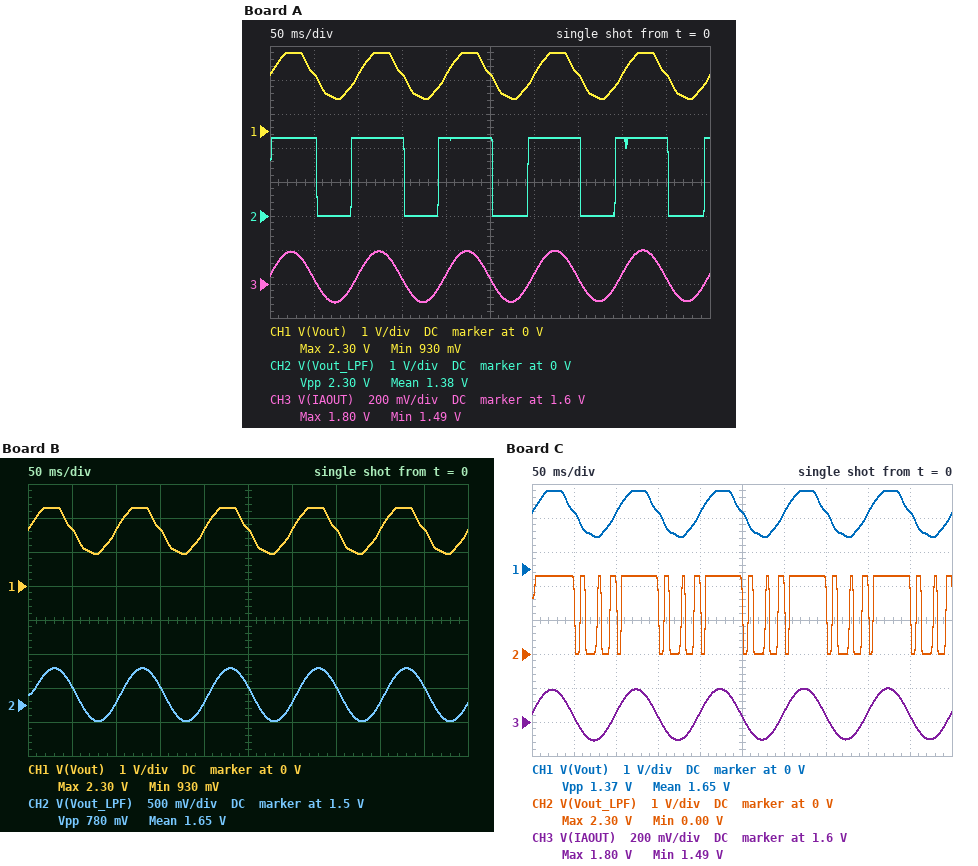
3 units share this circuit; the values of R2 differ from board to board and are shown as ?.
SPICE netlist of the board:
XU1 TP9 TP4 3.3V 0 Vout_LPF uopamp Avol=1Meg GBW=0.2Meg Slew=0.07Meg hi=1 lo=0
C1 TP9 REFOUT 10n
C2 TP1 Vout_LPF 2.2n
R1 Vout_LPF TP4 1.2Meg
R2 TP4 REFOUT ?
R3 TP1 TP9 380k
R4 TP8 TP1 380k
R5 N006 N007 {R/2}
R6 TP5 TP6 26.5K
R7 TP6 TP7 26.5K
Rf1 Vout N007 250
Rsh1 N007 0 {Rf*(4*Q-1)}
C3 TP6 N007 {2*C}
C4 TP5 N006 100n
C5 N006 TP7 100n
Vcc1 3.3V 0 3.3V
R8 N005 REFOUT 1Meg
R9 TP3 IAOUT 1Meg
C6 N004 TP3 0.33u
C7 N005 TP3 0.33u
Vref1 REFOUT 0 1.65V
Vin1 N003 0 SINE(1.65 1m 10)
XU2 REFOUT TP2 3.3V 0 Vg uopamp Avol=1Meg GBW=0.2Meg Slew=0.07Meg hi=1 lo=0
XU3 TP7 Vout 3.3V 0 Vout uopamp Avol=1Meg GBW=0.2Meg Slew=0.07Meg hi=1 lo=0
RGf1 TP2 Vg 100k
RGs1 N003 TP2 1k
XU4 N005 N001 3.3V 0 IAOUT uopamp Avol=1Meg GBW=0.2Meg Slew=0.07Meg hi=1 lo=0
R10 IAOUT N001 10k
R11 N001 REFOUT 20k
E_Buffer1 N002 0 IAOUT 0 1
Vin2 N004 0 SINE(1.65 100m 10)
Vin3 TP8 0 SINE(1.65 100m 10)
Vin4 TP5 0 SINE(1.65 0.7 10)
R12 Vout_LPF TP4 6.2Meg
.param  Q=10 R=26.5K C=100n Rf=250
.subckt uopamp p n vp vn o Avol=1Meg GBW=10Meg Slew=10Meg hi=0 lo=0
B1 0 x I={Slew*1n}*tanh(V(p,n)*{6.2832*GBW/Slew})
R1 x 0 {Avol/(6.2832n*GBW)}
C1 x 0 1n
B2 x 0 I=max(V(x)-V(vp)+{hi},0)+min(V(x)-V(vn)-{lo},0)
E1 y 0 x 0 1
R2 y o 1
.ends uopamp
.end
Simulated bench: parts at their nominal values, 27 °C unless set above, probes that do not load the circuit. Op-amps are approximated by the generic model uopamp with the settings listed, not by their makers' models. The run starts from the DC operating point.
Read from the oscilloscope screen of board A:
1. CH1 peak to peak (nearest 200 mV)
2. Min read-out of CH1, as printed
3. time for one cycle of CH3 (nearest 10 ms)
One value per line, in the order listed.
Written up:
1.4 V
930 mV
100 ms
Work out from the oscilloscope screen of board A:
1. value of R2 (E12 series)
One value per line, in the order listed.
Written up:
47 kΩ
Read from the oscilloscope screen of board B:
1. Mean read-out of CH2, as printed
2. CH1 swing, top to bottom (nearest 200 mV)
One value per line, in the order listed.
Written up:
1.65 V
1.4 V
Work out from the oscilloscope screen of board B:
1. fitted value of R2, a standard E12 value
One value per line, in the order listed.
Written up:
330 kΩ
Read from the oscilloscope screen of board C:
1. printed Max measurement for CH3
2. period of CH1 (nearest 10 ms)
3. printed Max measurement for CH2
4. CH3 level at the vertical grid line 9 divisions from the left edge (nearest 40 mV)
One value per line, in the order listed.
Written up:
1.80 V
100 ms
2.30 V
1.64 V
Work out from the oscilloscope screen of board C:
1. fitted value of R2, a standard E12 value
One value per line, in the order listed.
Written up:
82 kΩ
